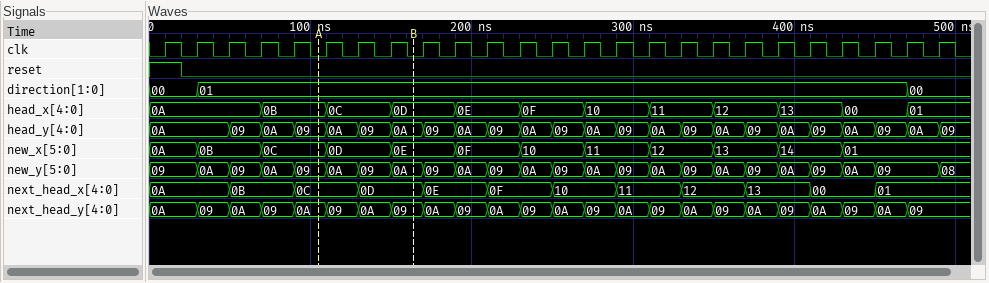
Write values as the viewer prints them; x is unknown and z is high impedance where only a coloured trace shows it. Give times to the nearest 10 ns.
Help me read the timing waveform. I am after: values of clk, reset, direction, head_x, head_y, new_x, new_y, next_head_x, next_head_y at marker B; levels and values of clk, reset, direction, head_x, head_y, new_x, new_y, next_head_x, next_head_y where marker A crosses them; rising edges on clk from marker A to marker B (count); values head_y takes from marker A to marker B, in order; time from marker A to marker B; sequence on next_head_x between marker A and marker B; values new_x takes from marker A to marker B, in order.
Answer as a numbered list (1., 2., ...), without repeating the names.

1. clk=0, reset=0, direction=01, head_x=0D, head_y=0A, new_x=0E, new_y=0A, next_head_x=0D, next_head_y=09
2. clk=0, reset=0, direction=01, head_x=0B, head_y=09, new_x=0C, new_y=09, next_head_x=0C, next_head_y=0A
3. 3
4. 09, 0A, 09, 0A
5. 60 ns
6. 0C, 0D
7. 0C, 0D, 0E
